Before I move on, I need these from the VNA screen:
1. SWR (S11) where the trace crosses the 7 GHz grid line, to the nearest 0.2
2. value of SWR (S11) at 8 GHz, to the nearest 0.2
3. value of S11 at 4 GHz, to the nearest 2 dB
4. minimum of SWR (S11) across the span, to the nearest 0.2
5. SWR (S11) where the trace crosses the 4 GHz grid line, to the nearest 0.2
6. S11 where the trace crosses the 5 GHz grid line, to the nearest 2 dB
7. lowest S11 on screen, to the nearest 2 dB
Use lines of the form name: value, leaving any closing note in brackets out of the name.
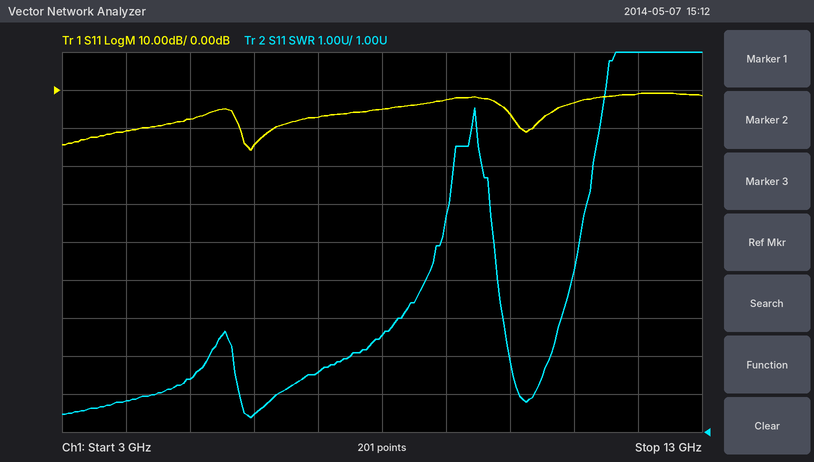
SWR (S11) where the trace crosses the 7 GHz grid line, to the nearest 0.2: 2.6
value of SWR (S11) at 8 GHz, to the nearest 0.2: 3.6
value of S11 at 4 GHz, to the nearest 2 dB: -10 dB
minimum of SWR (S11) across the span, to the nearest 0.2: 1.4
SWR (S11) where the trace crosses the 4 GHz grid line, to the nearest 0.2: 1.8
S11 where the trace crosses the 5 GHz grid line, to the nearest 2 dB: -8 dB
lowest S11 on screen, to the nearest 2 dB: -16 dB
